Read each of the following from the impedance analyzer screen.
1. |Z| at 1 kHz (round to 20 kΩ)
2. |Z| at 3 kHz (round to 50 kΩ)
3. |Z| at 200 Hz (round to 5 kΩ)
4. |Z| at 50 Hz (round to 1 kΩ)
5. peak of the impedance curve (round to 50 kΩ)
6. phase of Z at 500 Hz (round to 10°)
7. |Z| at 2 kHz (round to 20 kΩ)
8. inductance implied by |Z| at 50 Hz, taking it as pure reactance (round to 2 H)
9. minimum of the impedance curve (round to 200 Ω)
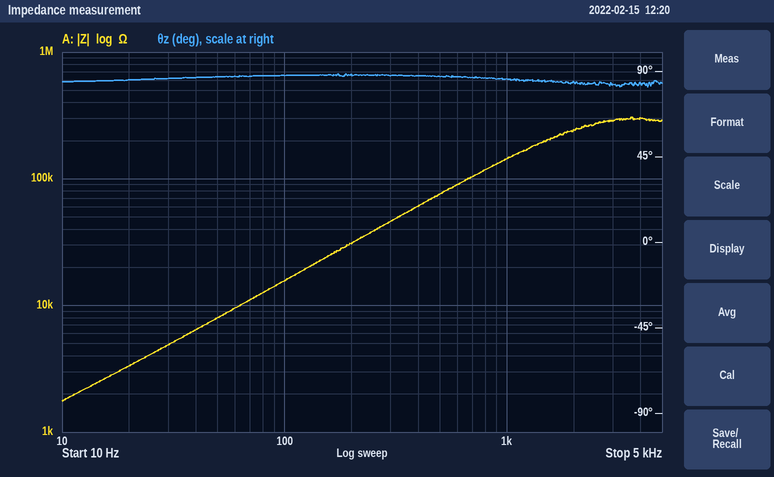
140 kΩ
300 kΩ
30 kΩ
8 kΩ
300 kΩ
90°
240 kΩ
26 H
1.8 kΩ
